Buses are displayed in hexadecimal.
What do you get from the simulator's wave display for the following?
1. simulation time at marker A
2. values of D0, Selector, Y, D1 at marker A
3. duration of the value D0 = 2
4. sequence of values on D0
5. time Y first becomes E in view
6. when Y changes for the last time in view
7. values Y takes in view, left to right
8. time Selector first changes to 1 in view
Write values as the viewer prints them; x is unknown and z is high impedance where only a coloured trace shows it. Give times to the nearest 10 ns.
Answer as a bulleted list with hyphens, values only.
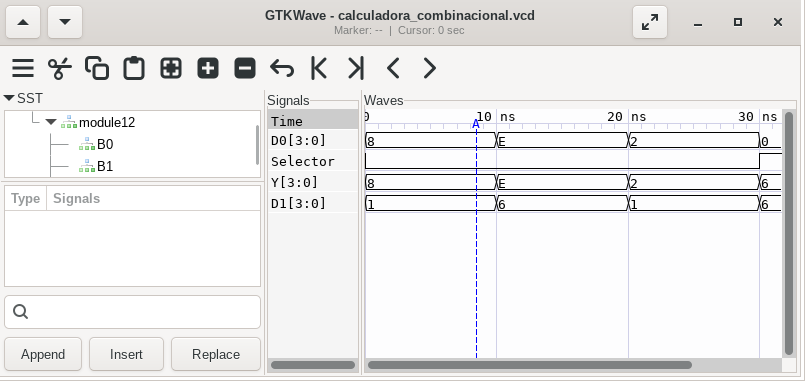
- 10 ns
- D0=8, Selector=0, Y=8, D1=1
- 10 ns
- 8, E, 2, 0
- 10 ns
- 30 ns
- 8, E, 2, 6
- 30 ns
